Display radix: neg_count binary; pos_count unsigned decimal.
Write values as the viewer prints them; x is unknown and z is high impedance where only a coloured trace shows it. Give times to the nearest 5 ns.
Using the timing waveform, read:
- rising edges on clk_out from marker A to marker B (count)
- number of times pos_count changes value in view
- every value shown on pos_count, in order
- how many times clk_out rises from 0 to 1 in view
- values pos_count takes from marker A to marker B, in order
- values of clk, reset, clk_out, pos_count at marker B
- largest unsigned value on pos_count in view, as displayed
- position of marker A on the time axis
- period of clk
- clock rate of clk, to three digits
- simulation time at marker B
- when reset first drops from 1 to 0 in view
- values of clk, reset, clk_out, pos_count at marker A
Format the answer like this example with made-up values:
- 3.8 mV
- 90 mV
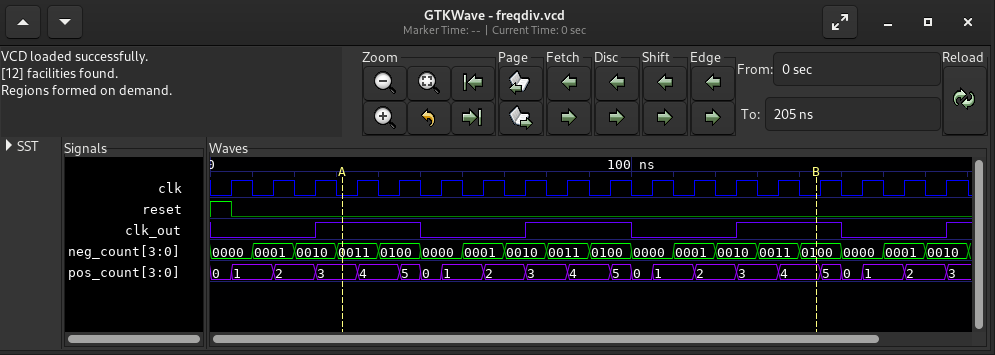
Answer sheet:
- 2
- 21
- 0, 1, 2, 3, 4, 5, 0, 1, 2, 3, 4, 5, 0, 1, 2, 3, 4, 5, 0, 1, 2, 3
- 4
- 3, 4, 5, 0, 1, 2, 3, 4, 5, 0, 1, 2, 3, 4
- clk=0, reset=0, clk_out=1, pos_count=4
- 5
- 30 ns
- 10 ns
- 100 MHz
- 145 ns
- 5 ns
- clk=0, reset=0, clk_out=1, pos_count=3
